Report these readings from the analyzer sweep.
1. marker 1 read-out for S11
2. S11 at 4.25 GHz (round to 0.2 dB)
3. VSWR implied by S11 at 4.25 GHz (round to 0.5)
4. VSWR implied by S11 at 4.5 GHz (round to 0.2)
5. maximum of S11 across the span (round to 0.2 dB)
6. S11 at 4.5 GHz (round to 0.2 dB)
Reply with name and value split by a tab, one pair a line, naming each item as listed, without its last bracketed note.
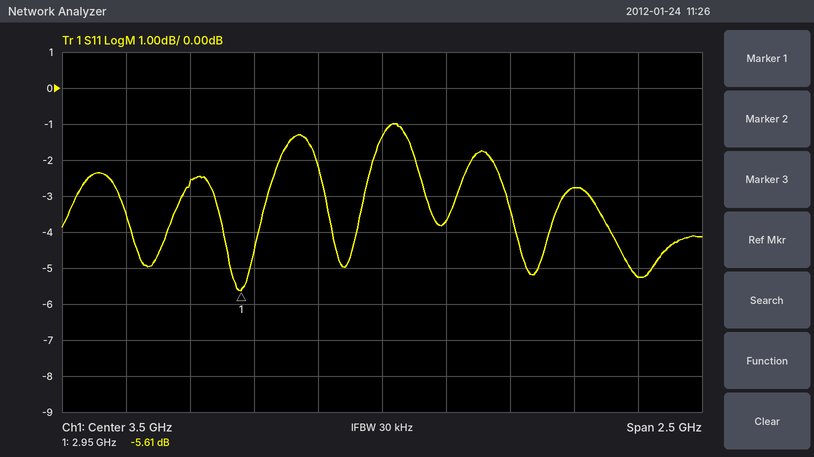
marker 1 read-out for S11	-5.61 dB
S11 at 4.25 GHz	-2.8 dB
VSWR implied by S11 at 4.25 GHz	6.5
VSWR implied by S11 at 4.5 GHz	3.4
maximum of S11 across the span	-1.0 dB
S11 at 4.5 GHz	-5.2 dB
